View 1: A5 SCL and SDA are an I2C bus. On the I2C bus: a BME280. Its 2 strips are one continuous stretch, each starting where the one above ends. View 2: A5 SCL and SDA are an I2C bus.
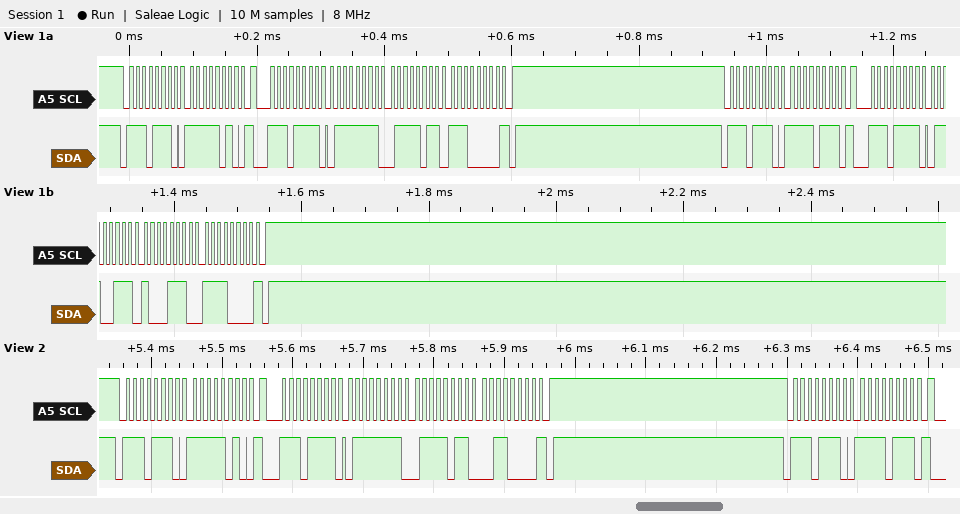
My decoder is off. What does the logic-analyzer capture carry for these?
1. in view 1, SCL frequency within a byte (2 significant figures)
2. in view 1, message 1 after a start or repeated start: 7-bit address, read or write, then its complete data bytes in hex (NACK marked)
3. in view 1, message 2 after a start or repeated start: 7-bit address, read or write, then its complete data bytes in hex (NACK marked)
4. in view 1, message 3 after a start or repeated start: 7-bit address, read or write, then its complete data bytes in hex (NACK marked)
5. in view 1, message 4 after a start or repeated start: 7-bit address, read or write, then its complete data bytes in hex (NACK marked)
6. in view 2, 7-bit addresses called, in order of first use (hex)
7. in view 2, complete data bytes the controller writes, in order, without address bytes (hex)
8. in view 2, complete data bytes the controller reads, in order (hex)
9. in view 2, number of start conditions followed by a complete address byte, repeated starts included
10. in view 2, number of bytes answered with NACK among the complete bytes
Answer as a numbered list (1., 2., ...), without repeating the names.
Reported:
1. 100 kHz
2. 0x77 write: FA
3. 0x77 read: 7F 7B E0 NACK
4. 0x77 write: F7
5. 0x77 read: 67 8E F0 NACK
6. 0x77
7. FA F7
8. 7F 7B 30
9. 3
10. 1
